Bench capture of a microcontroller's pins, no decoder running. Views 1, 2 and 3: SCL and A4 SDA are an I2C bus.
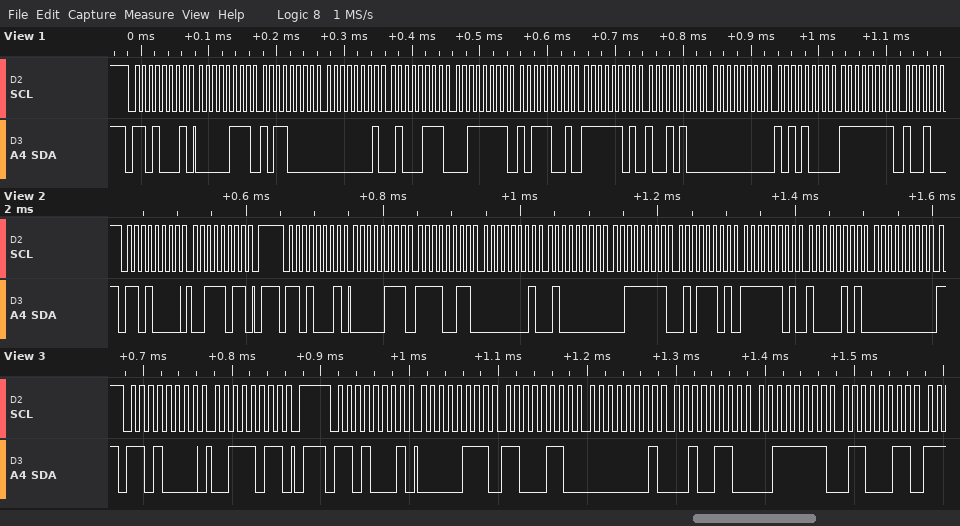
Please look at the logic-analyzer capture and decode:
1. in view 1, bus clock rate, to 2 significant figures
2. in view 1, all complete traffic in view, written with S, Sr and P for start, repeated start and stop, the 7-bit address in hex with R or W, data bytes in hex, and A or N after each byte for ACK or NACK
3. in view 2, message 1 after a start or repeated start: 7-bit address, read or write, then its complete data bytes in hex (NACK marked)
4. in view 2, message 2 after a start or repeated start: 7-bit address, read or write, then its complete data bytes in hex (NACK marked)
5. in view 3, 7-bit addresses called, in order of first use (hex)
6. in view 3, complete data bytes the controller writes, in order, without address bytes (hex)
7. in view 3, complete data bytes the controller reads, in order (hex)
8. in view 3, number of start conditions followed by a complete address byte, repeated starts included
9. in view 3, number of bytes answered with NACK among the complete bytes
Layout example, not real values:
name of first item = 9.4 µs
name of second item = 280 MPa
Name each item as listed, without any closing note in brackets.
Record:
in view 1, bus clock rate, to 2 significant figures = 100 kHz
in view 1, all complete traffic in view, written with S, Sr and P for start, repeated start and stop, the 7-bit address in hex with R or W, data bytes in hex, and A or N after each byte for ACK or NACK = S 68R A 07 A B0 A 01 A 47 A 3F A B9 A FD A 94 A 00 A A8 A FF A
in view 2, message 1 after a start or repeated start: 7-bit address, read or write, then its complete data bytes in hex = 0x68 write: 3B
in view 2, message 2 after a start or repeated start: 7-bit address, read or write, then its complete data bytes in hex = 0x68 read: 07 F3 01 40 3F 5D FD 85 00
in view 3, 7-bit addresses called, in order of first use = 0x68
in view 3, complete data bytes the controller writes, in order, without address bytes = 3B
in view 3, complete data bytes the controller reads, in order = 07 C6 01 26 3F 63
in view 3, number of start conditions followed by a complete address byte, repeated starts included = 2
in view 3, number of bytes answered with NACK among the complete bytes = 0
